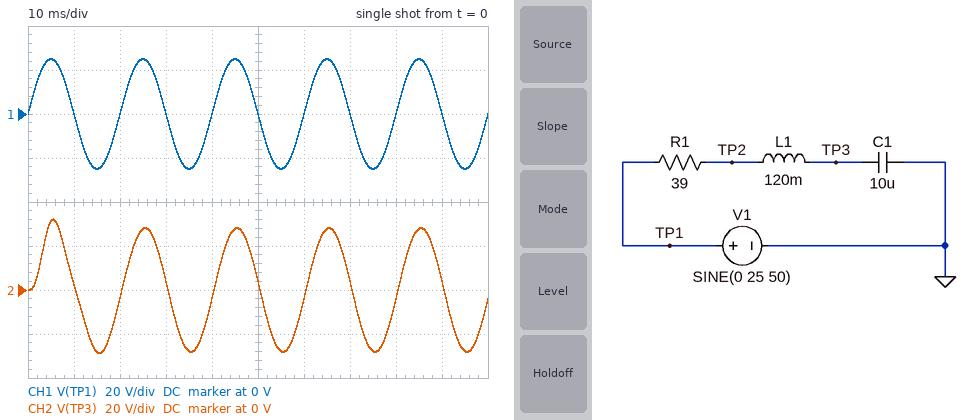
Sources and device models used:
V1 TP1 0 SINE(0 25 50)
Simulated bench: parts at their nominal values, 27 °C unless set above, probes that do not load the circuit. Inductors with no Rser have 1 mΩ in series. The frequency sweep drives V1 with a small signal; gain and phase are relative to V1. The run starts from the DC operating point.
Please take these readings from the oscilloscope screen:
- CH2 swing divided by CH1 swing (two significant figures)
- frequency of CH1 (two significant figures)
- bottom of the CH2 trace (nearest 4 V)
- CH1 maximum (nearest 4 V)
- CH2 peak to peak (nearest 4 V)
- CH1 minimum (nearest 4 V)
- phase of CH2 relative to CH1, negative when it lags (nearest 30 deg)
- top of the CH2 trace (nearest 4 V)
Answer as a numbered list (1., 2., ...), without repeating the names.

1. 1.2
2. 50 Hz
3. -28 V
4. 24 V
5. 60 V
6. -24 V
7. 0 deg
8. 32 V
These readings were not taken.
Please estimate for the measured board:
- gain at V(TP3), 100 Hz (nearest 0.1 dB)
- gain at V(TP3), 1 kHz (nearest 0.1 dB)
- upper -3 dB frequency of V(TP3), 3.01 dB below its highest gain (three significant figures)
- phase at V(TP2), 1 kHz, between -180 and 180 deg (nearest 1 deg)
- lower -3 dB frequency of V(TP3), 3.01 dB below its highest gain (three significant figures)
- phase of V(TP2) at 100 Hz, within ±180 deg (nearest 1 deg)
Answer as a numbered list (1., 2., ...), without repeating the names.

1. 4.7 dB
2. -33.3 dB
3. 165 Hz
4. 3 deg
5. 111 Hz
6. -25 deg
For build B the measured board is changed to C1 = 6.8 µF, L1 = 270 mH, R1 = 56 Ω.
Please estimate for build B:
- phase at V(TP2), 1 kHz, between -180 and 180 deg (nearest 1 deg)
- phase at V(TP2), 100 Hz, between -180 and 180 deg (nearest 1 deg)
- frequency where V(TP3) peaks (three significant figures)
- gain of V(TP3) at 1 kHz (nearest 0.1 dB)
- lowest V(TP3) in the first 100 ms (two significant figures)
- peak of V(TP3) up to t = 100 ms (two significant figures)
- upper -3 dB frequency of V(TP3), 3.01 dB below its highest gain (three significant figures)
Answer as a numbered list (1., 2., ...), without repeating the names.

1. 2 deg
2. -41 deg
3. 115 Hz
4. -37.1 dB
5. -30 V
6. 35 V
7. 131 Hz
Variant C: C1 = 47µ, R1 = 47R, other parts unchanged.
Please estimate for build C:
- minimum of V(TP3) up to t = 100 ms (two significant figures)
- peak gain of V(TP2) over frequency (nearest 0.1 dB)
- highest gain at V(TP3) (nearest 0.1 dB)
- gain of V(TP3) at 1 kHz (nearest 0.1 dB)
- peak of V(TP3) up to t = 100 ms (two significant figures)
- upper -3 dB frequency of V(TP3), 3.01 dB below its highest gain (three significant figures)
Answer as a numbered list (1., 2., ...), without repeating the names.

1. -30 V
2. 0 dB
3. 1.7 dB
4. -46.9 dB
5. 30 V
6. 79.0 Hz
